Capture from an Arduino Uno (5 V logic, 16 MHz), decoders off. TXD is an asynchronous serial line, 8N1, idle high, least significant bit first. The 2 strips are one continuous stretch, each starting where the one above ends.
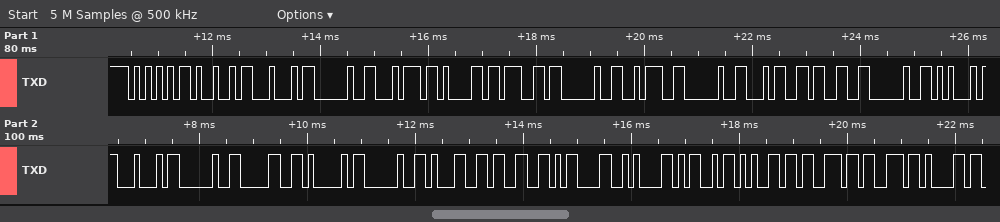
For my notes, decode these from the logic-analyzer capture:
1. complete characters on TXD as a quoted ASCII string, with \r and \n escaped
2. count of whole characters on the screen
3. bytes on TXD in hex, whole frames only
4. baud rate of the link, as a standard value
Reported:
"UID tag : 43 ED 0A 13\r\nMessa"
28
55 49 44 20 74 61 67 20 3A 20 34 33 20 45 44 20 30 41 20 31 33 0D 0A 4D 65 73 73 61
9600 baud
